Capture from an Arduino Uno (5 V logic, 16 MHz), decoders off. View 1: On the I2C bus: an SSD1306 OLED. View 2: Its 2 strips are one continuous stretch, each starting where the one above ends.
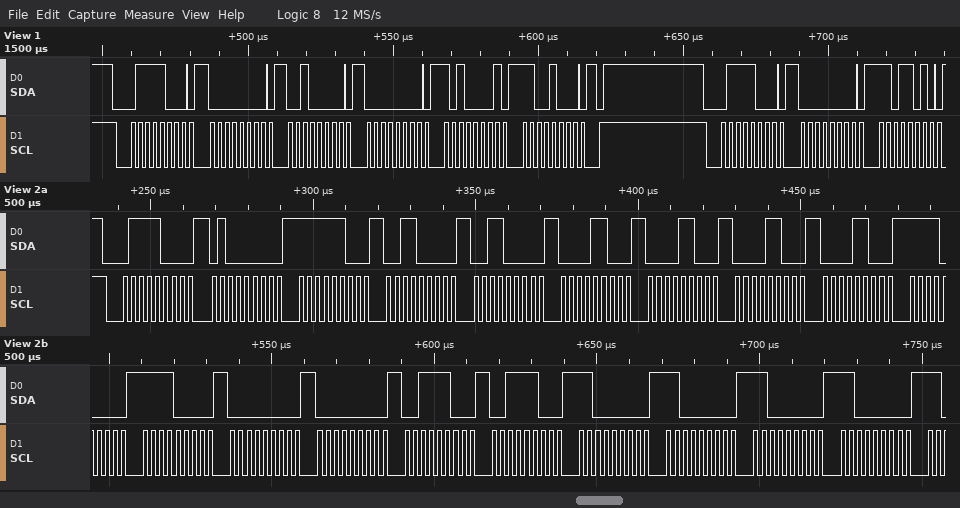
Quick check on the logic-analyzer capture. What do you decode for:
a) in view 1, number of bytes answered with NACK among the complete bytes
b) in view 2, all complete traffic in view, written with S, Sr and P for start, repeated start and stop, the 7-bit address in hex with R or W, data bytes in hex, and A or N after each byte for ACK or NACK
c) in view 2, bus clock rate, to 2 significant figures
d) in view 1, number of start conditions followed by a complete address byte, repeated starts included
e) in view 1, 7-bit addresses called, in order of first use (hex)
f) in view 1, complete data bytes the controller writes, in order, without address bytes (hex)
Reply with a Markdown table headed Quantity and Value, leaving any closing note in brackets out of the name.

| Quantity | Value |
|---|---|
| in view 1, number of bytes answered with NACK among the complete bytes | 0 |
| in view 2, all complete traffic in view, written with S, Sr and P for start, repeated start and stop, the 7-bit address in hex with R or W, data bytes in hex, and A or N after each byte for ACK or NACK | S 3CW A 40 A FC A 30 A 30 A 0C A 0C A 0C A 0C A F0 A F0 A 00 A 00 A 3C A 3C A C0 A C0 A C0 A C0 A |
| in view 2, bus clock rate, to 2 significant figures | 400 kHz |
| in view 1, number of start conditions followed by a complete address byte, repeated starts included | 2 |
| in view 1, 7-bit addresses called, in order of first use | 0x3C |
| in view 1, complete data bytes the controller writes, in order, without address bytes | 00 20 00 A1 C8 00 DA |
